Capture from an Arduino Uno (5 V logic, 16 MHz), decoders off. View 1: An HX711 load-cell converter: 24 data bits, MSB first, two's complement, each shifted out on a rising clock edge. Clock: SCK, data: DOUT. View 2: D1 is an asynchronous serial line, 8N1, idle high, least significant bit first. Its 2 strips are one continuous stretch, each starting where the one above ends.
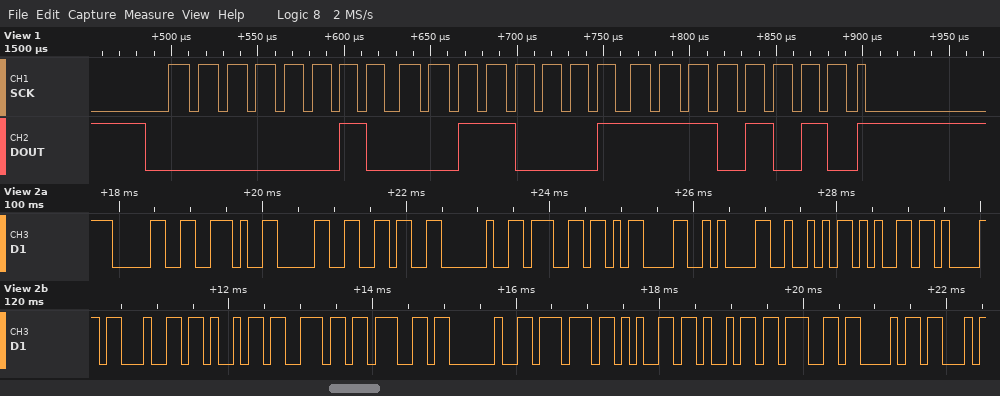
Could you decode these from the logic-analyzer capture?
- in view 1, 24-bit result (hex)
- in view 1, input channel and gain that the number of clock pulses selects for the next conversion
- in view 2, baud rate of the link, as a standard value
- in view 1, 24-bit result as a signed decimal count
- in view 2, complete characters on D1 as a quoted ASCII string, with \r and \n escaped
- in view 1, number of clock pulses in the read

0x0231EA
channel A, gain 128
9600 baud
143850
"0.06 g\r\nReading weigh"
25
